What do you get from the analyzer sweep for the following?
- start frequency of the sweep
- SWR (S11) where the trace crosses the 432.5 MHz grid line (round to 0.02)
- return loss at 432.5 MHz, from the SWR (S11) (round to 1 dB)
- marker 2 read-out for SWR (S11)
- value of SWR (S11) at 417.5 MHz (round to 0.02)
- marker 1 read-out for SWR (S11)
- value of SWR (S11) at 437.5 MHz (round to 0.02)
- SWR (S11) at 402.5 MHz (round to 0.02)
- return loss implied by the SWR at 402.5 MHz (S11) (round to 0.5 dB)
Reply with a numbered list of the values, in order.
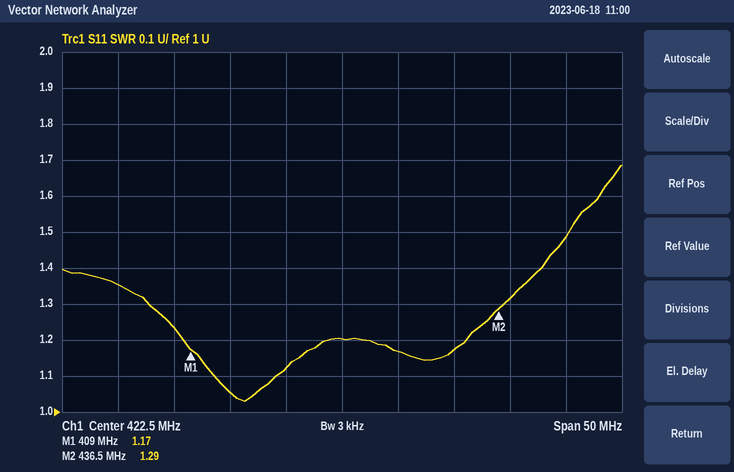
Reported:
1. 397.5 MHz
2. 1.18
3. 22 dB
4. 1.29
5. 1.12
6. 1.17
7. 1.32
8. 1.36
9. 16.5 dB
